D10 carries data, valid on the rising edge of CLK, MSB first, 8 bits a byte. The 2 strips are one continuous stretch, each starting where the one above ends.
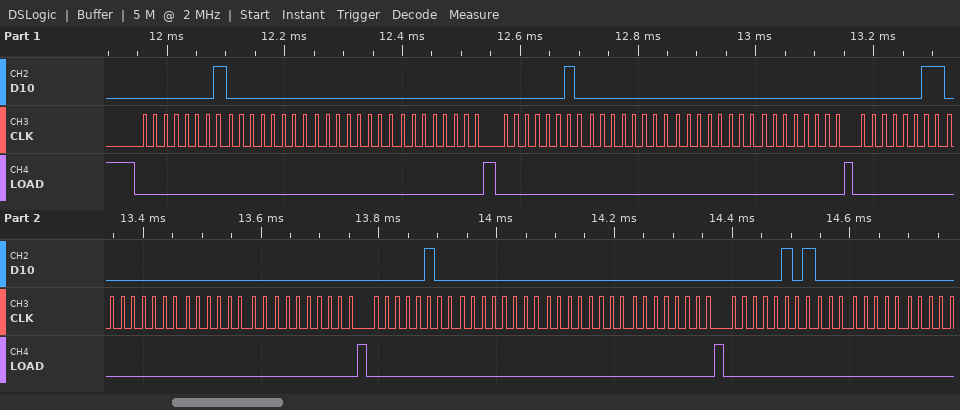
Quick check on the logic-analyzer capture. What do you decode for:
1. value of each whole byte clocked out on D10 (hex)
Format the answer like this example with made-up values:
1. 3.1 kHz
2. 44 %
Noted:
1. 01 00 00 00 02 00 00 00 03 00 00 00 04 00 00 00 05 00
